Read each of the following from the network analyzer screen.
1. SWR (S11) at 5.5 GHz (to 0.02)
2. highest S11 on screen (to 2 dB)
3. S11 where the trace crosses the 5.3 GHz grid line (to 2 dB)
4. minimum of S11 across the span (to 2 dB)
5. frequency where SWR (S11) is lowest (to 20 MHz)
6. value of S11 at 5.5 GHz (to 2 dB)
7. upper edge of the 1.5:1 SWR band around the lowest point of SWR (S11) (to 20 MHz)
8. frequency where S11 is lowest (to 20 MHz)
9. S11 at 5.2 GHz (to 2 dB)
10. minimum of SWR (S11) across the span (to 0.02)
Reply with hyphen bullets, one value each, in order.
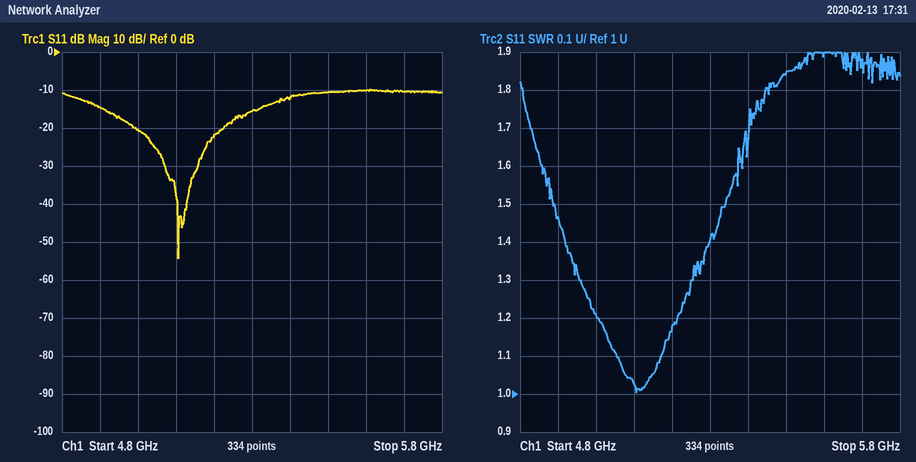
- 1.84
- -10 dB
- -16 dB
- -54 dB
- 5.10 GHz
- -10 dB
- 5.34 GHz
- 5.10 GHz
- -22 dB
- 1.00
